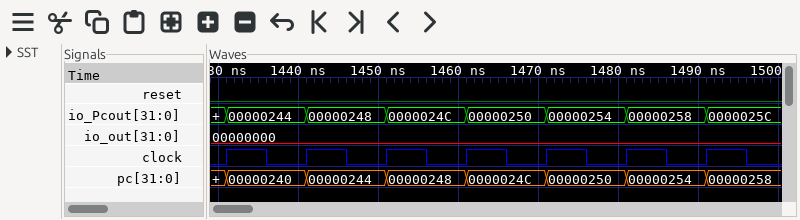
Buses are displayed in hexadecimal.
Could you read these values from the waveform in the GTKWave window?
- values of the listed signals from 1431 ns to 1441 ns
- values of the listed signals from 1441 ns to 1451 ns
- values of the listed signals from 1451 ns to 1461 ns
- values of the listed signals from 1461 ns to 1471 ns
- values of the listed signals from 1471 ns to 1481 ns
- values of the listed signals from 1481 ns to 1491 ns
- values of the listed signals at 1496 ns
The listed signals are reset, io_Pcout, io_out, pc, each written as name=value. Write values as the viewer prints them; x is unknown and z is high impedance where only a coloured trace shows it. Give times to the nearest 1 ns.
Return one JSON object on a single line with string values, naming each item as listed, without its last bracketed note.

{"values of the listed signals from 1431 ns to 1441 ns": "reset=0, io_Pcout=00000244, io_out=00000000, pc=00000240", "values of the listed signals from 1441 ns to 1451 ns": "reset=0, io_Pcout=00000248, io_out=00000000, pc=00000244", "values of the listed signals from 1451 ns to 1461 ns": "reset=0, io_Pcout=0000024C, io_out=00000000, pc=00000248", "values of the listed signals from 1461 ns to 1471 ns": "reset=0, io_Pcout=00000250, io_out=00000000, pc=0000024C", "values of the listed signals from 1471 ns to 1481 ns": "reset=0, io_Pcout=00000254, io_out=00000000, pc=00000250", "values of the listed signals from 1481 ns to 1491 ns": "reset=0, io_Pcout=00000258, io_out=00000000, pc=00000254", "values of the listed signals at 1496 ns": "reset=0, io_Pcout=0000025C, io_out=00000000, pc=00000258"}
